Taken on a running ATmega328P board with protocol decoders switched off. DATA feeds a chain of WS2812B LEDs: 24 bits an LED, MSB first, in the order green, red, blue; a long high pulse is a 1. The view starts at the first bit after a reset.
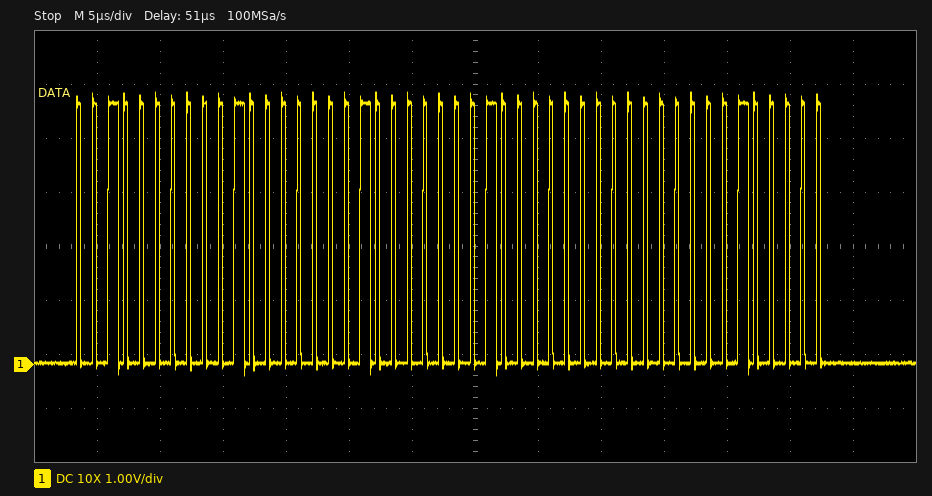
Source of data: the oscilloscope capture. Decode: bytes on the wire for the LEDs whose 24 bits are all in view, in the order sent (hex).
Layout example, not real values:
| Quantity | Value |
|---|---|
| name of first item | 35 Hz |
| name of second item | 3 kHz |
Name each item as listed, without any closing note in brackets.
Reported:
| Quantity | Value |
|---|---|
| bytes on the wire for the LEDs whose 24 bits are all in view, in the order sent | 20 20 20 20 00 20 |
